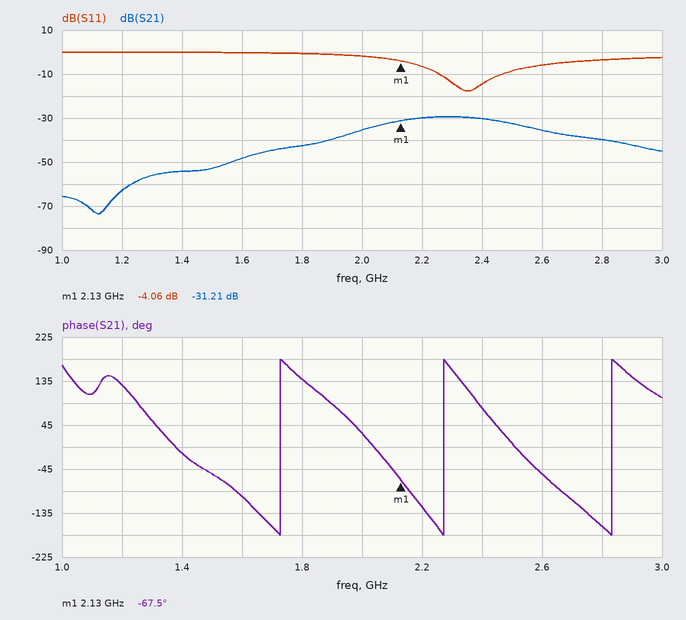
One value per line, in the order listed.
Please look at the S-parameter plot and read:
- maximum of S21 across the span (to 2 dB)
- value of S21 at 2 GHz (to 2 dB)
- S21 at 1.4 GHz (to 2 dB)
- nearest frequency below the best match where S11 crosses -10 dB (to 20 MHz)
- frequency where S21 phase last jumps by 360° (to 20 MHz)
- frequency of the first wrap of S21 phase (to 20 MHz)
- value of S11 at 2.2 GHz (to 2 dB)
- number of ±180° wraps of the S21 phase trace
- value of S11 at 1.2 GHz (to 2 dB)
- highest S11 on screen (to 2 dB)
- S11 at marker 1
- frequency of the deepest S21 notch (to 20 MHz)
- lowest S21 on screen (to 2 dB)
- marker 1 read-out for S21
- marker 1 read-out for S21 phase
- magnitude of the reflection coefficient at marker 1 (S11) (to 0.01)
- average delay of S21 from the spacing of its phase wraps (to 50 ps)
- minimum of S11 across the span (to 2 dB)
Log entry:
-30 dB
-36 dB
-54 dB
2.26 GHz
2.84 GHz
1.72 GHz
-6 dB
3
0 dB
0 dB
-4.06 dB
1.12 GHz
-74 dB
-31.21 dB
-67.5°
0.63
1.80 ns
-18 dB
